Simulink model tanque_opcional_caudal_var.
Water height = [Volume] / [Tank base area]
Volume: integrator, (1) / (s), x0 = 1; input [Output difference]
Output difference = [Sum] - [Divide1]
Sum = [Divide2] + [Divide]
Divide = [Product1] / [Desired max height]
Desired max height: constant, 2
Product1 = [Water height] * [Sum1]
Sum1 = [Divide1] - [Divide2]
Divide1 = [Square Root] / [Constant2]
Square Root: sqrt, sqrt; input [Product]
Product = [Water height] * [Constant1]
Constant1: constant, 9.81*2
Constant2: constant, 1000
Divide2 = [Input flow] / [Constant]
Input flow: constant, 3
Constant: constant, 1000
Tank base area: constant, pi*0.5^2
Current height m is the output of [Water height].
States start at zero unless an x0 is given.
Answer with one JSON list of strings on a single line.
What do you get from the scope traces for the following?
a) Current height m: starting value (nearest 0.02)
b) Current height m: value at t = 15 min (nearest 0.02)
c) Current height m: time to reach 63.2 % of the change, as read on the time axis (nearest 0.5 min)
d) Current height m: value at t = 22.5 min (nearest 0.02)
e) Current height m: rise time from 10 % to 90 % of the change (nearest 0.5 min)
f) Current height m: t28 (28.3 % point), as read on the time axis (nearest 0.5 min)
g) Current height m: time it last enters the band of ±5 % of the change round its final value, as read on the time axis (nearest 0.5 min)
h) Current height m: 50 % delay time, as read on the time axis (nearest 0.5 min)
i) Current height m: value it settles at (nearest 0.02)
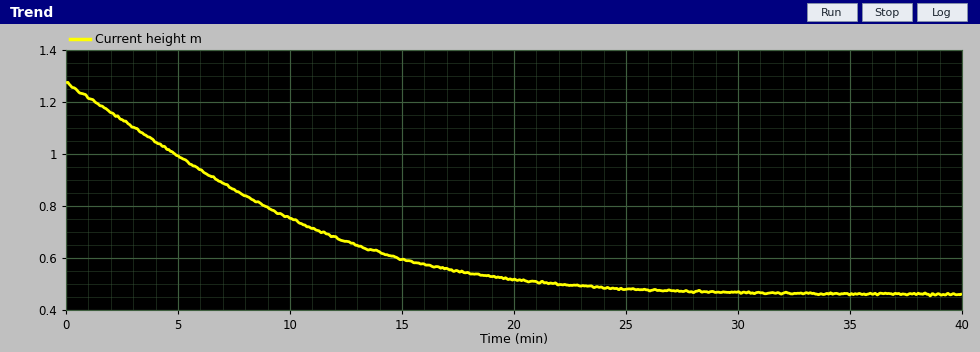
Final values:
["1.28", "0.60", "10.0 min", "0.50", "16.5 min", "4.0 min", "22.0 min", "7.5 min", "0.46"]
